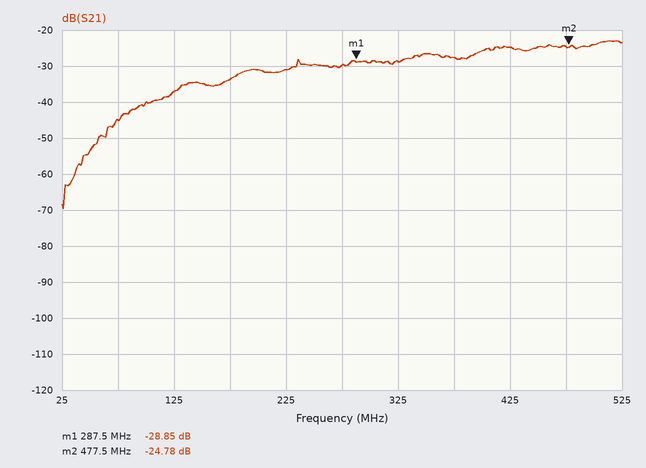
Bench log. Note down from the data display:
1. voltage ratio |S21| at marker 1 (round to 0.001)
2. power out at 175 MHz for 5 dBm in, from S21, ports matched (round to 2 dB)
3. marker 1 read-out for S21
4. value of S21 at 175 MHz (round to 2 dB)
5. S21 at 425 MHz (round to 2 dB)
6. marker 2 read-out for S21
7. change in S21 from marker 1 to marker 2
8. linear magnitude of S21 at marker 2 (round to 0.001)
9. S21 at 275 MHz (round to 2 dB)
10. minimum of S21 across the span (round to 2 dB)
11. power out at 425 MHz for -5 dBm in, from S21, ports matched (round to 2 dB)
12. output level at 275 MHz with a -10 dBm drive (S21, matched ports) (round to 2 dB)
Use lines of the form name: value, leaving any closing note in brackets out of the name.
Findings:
voltage ratio |S21| at marker 1: 0.036
power out at 175 MHz for 5 dBm in, from S21, ports matched: -28 dBm
marker 1 read-out for S21: -28.85 dB
value of S21 at 175 MHz: -34 dB
S21 at 425 MHz: -24 dB
marker 2 read-out for S21: -24.78 dB
change in S21 from marker 1 to marker 2: 4.07 dB
linear magnitude of S21 at marker 2: 0.058
S21 at 275 MHz: -30 dB
minimum of S21 across the span: -70 dB
power out at 425 MHz for -5 dBm in, from S21, ports matched: -30 dBm
output level at 275 MHz with a -10 dBm drive (S21, matched ports): -40 dBm
